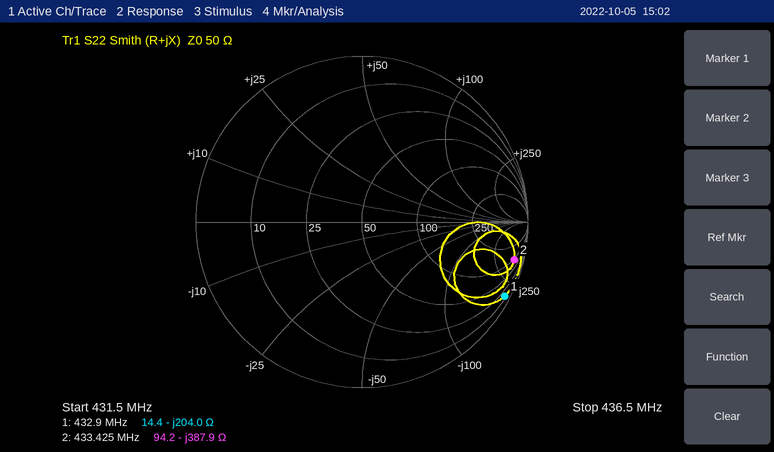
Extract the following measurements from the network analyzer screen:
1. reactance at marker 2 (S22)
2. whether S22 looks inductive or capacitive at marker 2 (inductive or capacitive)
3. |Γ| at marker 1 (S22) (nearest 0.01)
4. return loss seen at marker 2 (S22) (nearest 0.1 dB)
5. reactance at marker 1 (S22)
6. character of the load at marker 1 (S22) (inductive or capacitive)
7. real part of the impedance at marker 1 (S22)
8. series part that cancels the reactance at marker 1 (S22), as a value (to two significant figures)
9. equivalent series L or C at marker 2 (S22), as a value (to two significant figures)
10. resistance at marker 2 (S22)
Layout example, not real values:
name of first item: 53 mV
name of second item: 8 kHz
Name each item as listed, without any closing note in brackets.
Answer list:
reactance at marker 2: -387.9 Ω
whether S22 looks inductive or capacitive at marker 2: capacitive
|Γ| at marker 1 (S22): 0.97
return loss seen at marker 2 (S22): 0.5 dB
reactance at marker 1: -204.0 Ω
character of the load at marker 1 (S22): capacitive
real part of the impedance at marker 1: 14.4 Ω
series part that cancels the reactance at marker 1 (S22), as a value: 75 nH
equivalent series L or C at marker 2 (S22), as a value: 950 fF
resistance at marker 2: 94.2 Ω
